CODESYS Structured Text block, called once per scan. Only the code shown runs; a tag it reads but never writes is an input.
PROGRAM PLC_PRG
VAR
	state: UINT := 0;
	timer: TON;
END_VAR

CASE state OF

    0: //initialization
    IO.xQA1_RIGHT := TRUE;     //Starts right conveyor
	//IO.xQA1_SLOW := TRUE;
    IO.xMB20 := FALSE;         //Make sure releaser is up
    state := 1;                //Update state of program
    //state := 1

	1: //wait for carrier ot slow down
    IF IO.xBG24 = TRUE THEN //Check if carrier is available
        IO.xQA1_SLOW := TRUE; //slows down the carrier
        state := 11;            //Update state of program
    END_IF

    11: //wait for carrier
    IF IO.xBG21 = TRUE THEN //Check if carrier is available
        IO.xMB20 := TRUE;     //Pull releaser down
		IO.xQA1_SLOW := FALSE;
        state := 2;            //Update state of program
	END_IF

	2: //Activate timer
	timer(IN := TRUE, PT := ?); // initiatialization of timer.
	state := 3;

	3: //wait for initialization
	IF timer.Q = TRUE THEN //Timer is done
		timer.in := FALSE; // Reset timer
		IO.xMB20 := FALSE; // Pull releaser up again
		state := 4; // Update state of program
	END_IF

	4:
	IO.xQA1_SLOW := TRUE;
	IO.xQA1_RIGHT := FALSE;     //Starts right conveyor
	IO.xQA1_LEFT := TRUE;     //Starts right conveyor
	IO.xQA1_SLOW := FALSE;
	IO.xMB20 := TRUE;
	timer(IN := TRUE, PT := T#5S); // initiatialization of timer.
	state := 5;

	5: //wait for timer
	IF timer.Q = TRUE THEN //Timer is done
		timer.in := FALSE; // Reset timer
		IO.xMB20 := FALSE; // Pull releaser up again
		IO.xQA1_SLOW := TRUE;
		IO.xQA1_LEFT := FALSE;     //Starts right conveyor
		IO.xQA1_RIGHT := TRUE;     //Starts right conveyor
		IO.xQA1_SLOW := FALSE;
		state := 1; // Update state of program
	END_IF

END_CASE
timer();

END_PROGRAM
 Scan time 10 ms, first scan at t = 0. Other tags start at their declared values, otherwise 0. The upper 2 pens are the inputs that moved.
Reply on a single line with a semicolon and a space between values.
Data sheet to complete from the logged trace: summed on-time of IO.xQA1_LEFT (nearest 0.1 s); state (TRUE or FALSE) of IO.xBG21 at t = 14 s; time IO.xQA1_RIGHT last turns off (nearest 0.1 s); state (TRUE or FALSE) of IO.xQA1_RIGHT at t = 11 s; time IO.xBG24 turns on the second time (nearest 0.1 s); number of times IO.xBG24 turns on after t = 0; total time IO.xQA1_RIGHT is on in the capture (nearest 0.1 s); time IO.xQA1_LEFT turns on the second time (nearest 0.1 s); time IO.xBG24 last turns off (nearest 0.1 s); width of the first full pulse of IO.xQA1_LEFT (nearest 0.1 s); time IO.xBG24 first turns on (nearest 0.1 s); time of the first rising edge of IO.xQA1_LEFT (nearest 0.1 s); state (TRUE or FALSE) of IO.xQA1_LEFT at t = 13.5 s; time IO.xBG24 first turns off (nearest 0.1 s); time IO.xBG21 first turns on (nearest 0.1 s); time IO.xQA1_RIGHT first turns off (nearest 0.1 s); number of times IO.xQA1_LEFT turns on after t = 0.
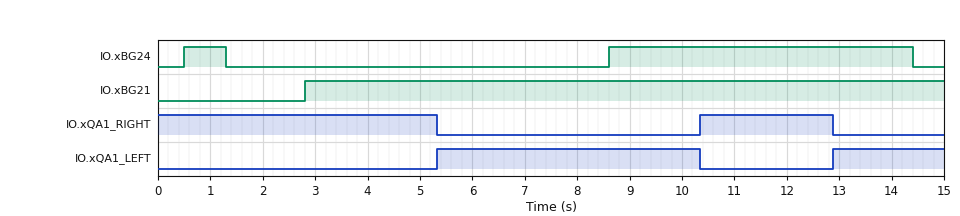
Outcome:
7.1 s; TRUE; 12.9 s; TRUE; 8.6 s; 2; 7.9 s; 12.9 s; 14.4 s; 5.0 s; 0.5 s; 5.3 s; TRUE; 1.3 s; 2.8 s; 5.3 s; 2
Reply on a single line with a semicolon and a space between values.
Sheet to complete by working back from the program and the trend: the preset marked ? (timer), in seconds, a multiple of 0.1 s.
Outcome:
2.5 s
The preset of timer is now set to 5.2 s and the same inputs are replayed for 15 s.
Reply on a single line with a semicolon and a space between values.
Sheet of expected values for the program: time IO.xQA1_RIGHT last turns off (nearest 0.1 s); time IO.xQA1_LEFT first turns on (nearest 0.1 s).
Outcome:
8.0 s; 8.0 s
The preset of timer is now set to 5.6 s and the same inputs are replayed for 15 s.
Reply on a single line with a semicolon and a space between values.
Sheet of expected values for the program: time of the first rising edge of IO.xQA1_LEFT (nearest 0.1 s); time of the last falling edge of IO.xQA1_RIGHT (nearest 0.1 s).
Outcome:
8.4 s; 8.4 s
